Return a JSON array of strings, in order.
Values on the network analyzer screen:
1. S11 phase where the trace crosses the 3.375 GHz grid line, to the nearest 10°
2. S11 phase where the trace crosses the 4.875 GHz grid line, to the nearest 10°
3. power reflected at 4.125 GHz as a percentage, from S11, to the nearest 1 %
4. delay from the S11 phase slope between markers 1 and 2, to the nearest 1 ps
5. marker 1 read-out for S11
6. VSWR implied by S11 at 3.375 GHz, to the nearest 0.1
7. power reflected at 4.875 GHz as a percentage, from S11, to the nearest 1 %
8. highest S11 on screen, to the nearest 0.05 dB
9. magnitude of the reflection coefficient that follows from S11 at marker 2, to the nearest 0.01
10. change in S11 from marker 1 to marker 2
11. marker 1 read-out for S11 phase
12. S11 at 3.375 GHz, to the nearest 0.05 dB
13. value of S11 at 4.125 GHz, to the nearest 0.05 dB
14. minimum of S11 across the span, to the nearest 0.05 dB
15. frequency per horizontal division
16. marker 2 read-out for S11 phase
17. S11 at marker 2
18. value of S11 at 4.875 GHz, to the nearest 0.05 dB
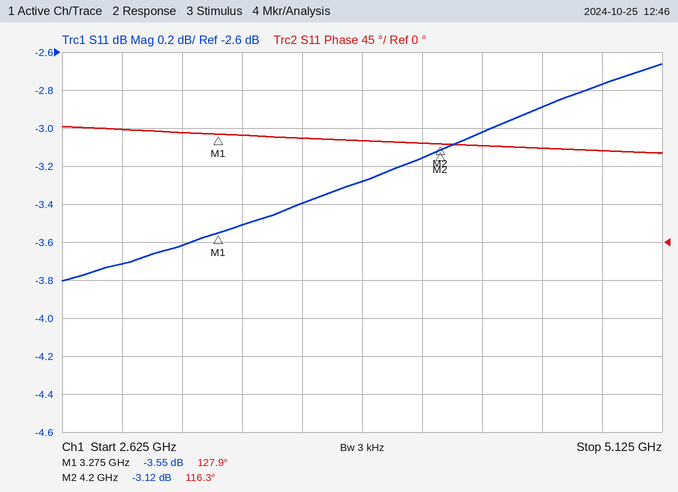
["130°", "110°", "48 %", "35 ps", "-3.55 dB", "5.0", "53 %", "-2.65 dB", "0.70", "0.43 dB", "127.9°", "-3.50 dB", "-3.15 dB", "-3.80 dB", "250 MHz", "116.3°", "-3.12 dB", "-2.75 dB"]
